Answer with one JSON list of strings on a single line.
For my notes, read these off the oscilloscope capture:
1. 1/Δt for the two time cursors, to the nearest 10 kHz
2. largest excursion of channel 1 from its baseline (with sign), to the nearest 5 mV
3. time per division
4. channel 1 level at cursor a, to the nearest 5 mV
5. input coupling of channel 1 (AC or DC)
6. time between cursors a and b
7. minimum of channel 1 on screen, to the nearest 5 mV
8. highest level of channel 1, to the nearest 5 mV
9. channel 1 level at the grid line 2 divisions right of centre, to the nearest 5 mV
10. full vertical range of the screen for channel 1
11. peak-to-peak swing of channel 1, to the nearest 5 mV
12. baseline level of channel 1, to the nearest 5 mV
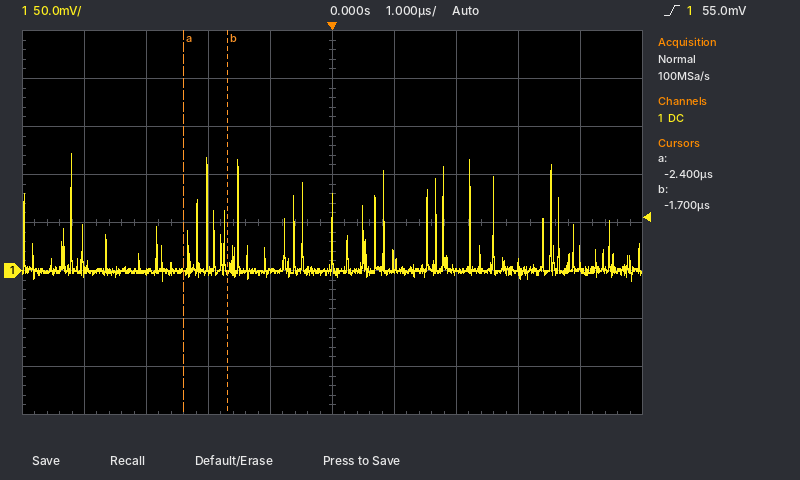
["1.43 MHz", "+120 mV", "1 µs", "0 mV", "DC", "700 ns", "-10 mV", "120 mV", "0 mV", "400 mV", "130 mV", "0 mV"]
